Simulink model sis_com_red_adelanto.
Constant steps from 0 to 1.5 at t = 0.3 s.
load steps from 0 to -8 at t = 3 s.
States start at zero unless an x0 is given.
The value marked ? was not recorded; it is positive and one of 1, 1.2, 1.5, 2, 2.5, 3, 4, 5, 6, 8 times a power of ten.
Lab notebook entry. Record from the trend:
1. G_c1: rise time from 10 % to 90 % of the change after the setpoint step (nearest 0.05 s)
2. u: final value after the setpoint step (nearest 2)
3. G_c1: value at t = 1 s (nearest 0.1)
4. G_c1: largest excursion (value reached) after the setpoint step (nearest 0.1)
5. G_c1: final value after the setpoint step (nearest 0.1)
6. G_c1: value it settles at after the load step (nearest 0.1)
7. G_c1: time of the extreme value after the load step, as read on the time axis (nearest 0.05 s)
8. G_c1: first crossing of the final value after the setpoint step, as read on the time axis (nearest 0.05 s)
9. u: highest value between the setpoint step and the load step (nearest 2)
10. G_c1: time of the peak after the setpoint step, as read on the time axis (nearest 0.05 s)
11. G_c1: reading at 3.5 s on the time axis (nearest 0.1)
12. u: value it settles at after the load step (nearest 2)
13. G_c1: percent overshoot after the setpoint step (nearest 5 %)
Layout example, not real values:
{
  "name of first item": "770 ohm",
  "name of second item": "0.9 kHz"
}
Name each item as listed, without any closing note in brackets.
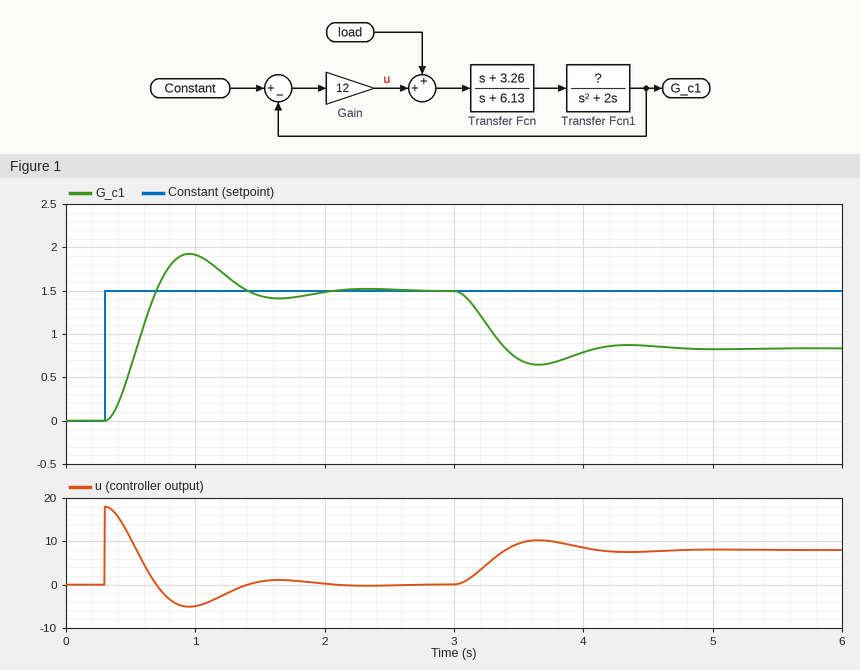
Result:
{
  "G_c1: rise time from 10 % to 90 % of the change after the setpoint step": "0.25 s",
  "u: final value after the setpoint step": "0",
  "G_c1: value at t = 1 s": "1.9",
  "G_c1: largest excursion (value reached) after the setpoint step": "1.9",
  "G_c1: final value after the setpoint step": "1.5",
  "G_c1: value it settles at after the load step": "0.8",
  "G_c1: time of the extreme value after the load step, as read on the time axis": "3.65 s",
  "G_c1: first crossing of the final value after the setpoint step, as read on the time axis": "0.70 s",
  "u: highest value between the setpoint step and the load step": "18",
  "G_c1: time of the peak after the setpoint step, as read on the time axis": "0.95 s",
  "G_c1: reading at 3.5 s on the time axis": "0.7",
  "u: value it settles at after the load step": "8",
  "G_c1: percent overshoot after the setpoint step": "30 %"
}
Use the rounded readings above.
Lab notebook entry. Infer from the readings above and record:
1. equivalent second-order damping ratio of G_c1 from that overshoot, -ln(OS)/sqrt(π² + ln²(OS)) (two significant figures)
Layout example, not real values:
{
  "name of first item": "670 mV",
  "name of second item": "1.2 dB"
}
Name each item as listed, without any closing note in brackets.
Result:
{
  "equivalent second-order damping ratio of G_c1 from that overshoot, -ln(OS)/sqrt(π² + ln²(OS))": "0.36"
}
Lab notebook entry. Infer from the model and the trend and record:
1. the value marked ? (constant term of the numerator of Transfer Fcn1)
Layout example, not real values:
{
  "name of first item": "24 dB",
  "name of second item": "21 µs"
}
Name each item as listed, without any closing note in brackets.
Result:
{
  "the value marked ?": "2.5"
}
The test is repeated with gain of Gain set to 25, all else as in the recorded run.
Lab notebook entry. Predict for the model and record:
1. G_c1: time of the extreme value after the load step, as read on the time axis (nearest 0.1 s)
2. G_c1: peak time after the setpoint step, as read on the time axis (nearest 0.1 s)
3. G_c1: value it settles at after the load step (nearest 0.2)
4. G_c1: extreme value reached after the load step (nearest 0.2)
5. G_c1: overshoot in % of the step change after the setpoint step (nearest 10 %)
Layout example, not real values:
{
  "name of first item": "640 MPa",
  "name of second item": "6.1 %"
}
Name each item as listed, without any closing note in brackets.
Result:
{
  "G_c1: time of the extreme value after the load step, as read on the time axis": "3.4 s",
  "G_c1: peak time after the setpoint step, as read on the time axis": "0.7 s",
  "G_c1: value it settles at after the load step": "1.2",
  "G_c1: extreme value reached after the load step": "1.0",
  "G_c1: overshoot in % of the step change after the setpoint step": "40 %"
}
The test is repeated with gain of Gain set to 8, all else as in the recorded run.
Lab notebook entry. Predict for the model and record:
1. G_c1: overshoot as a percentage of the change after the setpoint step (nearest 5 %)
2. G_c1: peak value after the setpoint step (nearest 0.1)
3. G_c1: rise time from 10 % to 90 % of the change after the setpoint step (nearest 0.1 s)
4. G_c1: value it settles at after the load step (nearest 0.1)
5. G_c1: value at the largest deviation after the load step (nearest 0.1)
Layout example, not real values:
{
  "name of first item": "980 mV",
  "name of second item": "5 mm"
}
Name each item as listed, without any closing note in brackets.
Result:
{
  "G_c1: overshoot as a percentage of the change after the setpoint step": "20 %",
  "G_c1: peak value after the setpoint step": "1.8",
  "G_c1: rise time from 10 % to 90 % of the change after the setpoint step": "0.4 s",
  "G_c1: value it settles at after the load step": "0.5",
  "G_c1: value at the largest deviation after the load step": "0.3"
}
